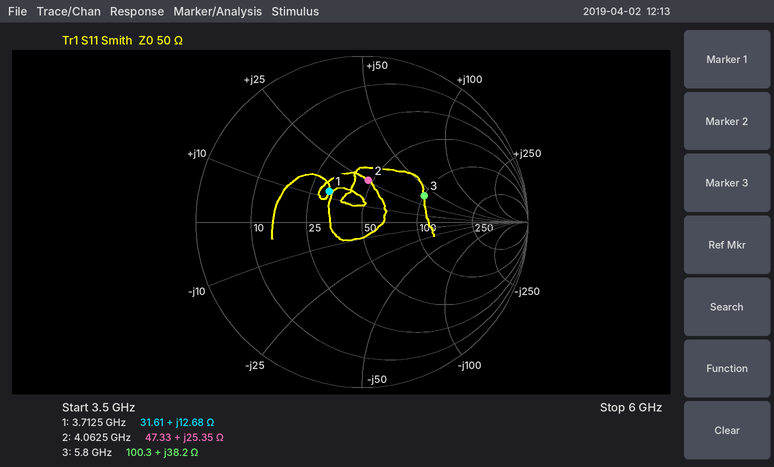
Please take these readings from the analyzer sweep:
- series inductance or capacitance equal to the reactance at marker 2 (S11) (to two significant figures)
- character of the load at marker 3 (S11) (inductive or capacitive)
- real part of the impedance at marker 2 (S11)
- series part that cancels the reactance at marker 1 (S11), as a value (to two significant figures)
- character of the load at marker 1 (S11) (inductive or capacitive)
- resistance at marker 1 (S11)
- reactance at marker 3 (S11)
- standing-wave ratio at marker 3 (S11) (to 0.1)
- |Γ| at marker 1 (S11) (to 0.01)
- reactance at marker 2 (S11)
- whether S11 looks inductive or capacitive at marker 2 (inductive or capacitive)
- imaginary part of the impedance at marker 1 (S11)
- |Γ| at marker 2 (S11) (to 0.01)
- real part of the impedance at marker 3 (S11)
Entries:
990 pH
inductive
47.33 Ω
3.4 pF
inductive
31.61 Ω
+38.2 Ω
2.4
0.27
+25.35 Ω
inductive
+12.68 Ω
0.25
100.3 Ω
